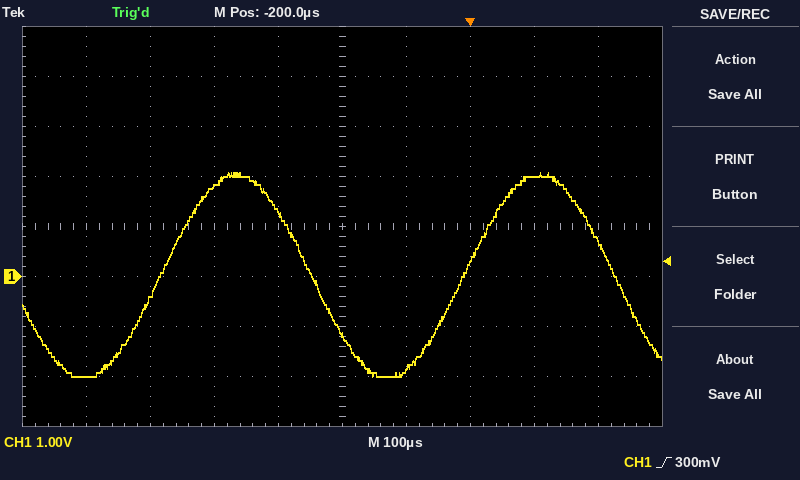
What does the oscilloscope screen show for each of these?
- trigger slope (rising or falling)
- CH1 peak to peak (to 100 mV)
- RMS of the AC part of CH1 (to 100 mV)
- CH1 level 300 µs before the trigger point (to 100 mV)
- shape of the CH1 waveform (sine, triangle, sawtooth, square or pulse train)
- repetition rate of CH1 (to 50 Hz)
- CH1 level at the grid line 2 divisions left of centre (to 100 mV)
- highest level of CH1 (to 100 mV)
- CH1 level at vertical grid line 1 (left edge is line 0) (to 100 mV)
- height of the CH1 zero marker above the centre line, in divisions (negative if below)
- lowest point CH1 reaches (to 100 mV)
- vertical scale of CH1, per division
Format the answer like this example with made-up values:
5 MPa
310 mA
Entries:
rising
4.1 V
1.4 V
1.3 V
sine
2.10 kHz
1.8 V
2.1 V
-2.0 V
-1.0 div
-2.0 V
1 V
